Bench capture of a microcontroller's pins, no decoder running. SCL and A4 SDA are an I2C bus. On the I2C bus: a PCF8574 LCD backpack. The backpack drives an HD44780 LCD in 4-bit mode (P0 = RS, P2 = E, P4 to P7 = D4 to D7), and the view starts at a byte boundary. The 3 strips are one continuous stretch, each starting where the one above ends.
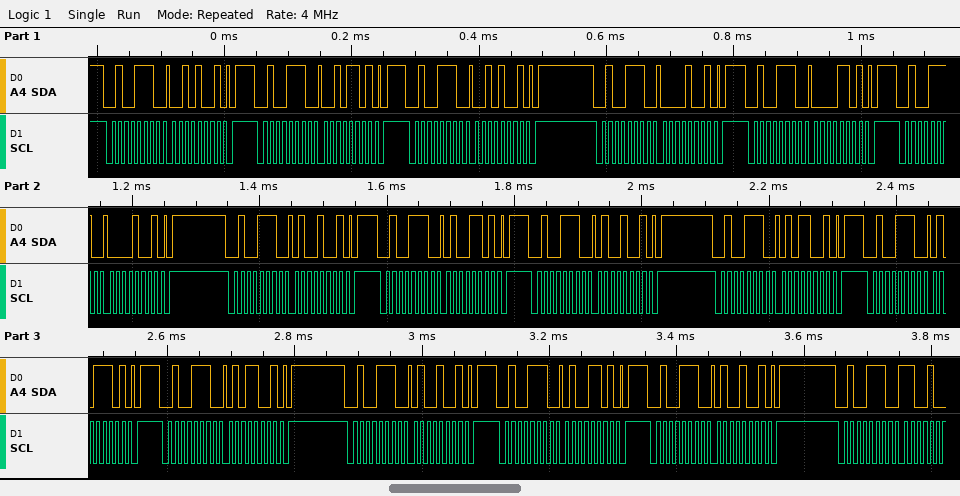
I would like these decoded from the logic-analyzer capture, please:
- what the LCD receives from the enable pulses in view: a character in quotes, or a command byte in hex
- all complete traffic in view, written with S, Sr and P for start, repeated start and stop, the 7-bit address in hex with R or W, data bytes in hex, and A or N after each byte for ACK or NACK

' ' 'E'
S 27W A 29 A P S 27W A 2D A P S 27W A 29 A P S 27W A 09 A P S 27W A 0D A P S 27W A 09 A P S 27W A 49 A P S 27W A 4D A P S 27W A 49 A P S 27W A 59 A P S 27W A 5D A P S 27W A 59 A P S 27W A 49 A P S 27W A 4D A P S 27W A 49 A P S 27W A
